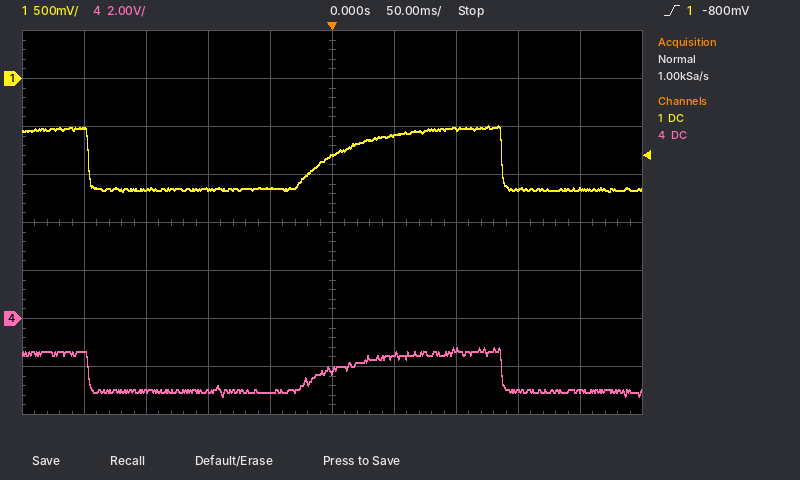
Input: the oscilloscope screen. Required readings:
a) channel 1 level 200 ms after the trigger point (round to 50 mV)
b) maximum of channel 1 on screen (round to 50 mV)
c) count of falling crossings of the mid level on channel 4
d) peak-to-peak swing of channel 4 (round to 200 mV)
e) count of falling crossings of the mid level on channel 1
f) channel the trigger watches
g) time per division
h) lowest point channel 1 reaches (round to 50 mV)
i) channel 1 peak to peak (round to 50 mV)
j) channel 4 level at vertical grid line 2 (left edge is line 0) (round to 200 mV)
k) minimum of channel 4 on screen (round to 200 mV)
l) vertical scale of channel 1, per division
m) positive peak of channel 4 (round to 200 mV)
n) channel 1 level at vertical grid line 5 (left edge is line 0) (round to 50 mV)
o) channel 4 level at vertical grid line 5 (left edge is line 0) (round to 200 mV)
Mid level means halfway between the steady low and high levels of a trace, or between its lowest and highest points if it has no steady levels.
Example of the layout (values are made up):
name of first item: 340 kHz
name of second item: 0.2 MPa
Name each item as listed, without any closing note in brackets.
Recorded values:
channel 1 level 200 ms after the trigger point: -1.15 V
maximum of channel 1 on screen: -500 mV
count of falling crossings of the mid level on channel 4: 2
peak-to-peak swing of channel 4: 2.0 V
count of falling crossings of the mid level on channel 1: 2
channel the trigger watches: channel 1
time per division: 50 ms
lowest point channel 1 reaches: -1.20 V
channel 1 peak to peak: 700 mV
channel 4 level at vertical grid line 2 (left edge is line 0): -3.0 V
minimum of channel 4 on screen: -3.2 V
vertical scale of channel 1, per division: 500 mV
positive peak of channel 4: -1.2 V
channel 1 level at vertical grid line 5 (left edge is line 0): -800 mV
channel 4 level at vertical grid line 5 (left edge is line 0): -2.2 V
